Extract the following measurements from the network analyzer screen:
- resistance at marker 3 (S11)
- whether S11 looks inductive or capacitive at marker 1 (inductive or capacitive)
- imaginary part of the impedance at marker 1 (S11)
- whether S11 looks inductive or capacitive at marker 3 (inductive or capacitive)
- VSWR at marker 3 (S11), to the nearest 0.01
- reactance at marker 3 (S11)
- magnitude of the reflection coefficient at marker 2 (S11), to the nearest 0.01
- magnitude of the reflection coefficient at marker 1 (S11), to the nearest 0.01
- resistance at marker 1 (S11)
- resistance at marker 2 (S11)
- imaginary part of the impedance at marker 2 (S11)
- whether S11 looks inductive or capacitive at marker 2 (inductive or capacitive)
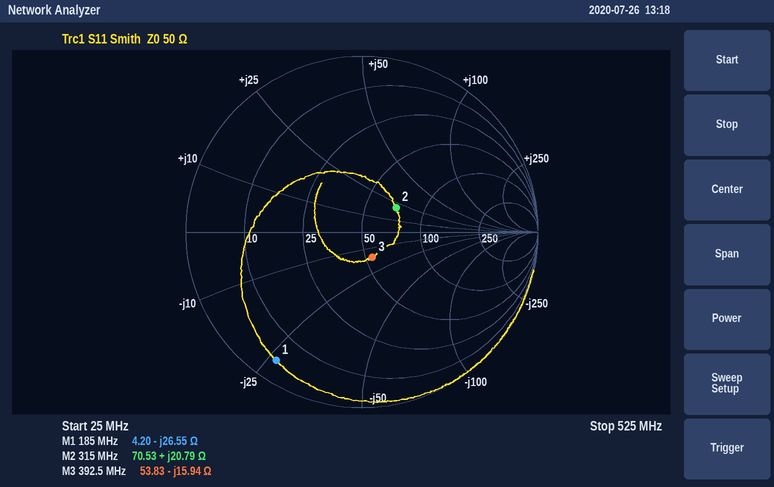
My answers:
53.83 Ω
capacitive
-26.55 Ω
capacitive
1.37
-15.94 Ω
0.24
0.88
4.20 Ω
70.53 Ω
+20.79 Ω
inductive
